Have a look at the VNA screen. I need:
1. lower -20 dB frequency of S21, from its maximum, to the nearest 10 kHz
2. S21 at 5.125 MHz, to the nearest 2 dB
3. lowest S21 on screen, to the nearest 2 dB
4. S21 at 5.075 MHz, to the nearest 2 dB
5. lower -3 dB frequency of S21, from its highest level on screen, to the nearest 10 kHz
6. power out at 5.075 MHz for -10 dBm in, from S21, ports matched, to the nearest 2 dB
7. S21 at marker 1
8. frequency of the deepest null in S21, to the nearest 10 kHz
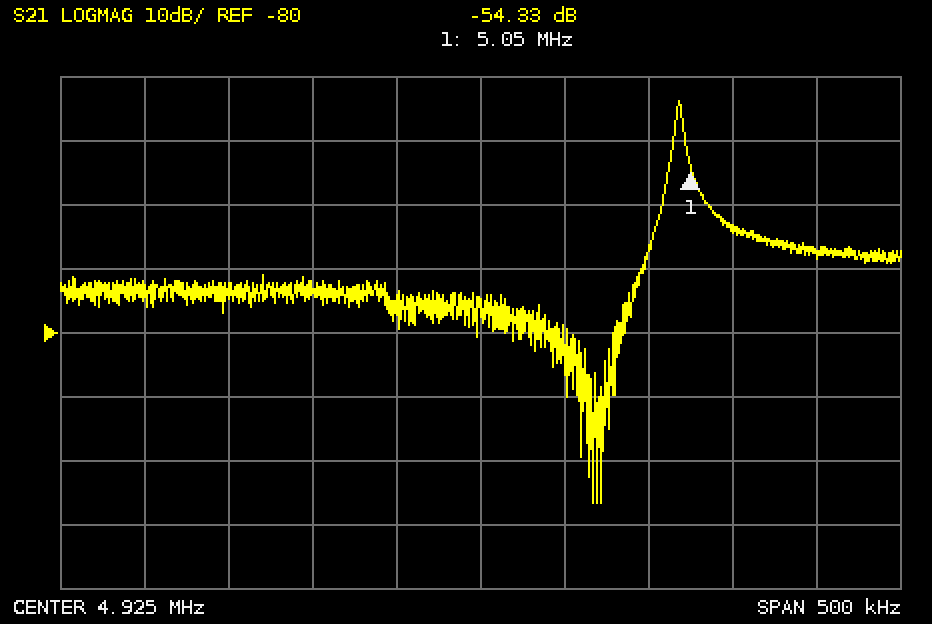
5.03 MHz
-68 dB
-106 dB
-64 dB
5.04 MHz
-74 dBm
-54.33 dB
4.99 MHz
